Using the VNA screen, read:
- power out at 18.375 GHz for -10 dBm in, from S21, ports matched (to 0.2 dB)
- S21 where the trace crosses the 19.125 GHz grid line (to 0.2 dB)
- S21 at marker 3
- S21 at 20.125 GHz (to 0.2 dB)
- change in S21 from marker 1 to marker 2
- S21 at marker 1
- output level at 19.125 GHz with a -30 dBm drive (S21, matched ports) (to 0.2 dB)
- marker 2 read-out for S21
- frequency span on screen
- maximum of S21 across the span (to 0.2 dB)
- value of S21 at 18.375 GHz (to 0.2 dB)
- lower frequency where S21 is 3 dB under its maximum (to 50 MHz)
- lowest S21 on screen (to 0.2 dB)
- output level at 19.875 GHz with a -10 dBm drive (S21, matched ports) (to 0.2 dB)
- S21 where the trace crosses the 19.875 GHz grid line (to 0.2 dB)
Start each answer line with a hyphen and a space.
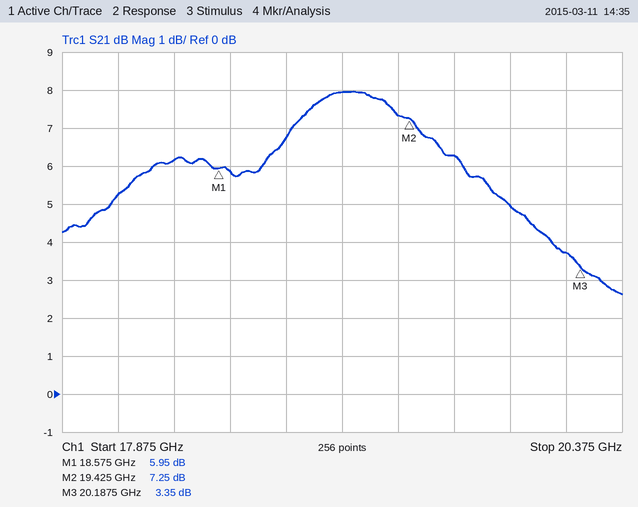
- -3.8 dBm
- 8.0 dB
- 3.35 dB
- 3.8 dB
- 1.30 dB
- 5.95 dB
- -22.0 dBm
- 7.25 dB
- 2.5 GHz
- 8.0 dB
- 6.2 dB
- 18.10 GHz
- 2.6 dB
- -5.0 dBm
- 5.0 dB
